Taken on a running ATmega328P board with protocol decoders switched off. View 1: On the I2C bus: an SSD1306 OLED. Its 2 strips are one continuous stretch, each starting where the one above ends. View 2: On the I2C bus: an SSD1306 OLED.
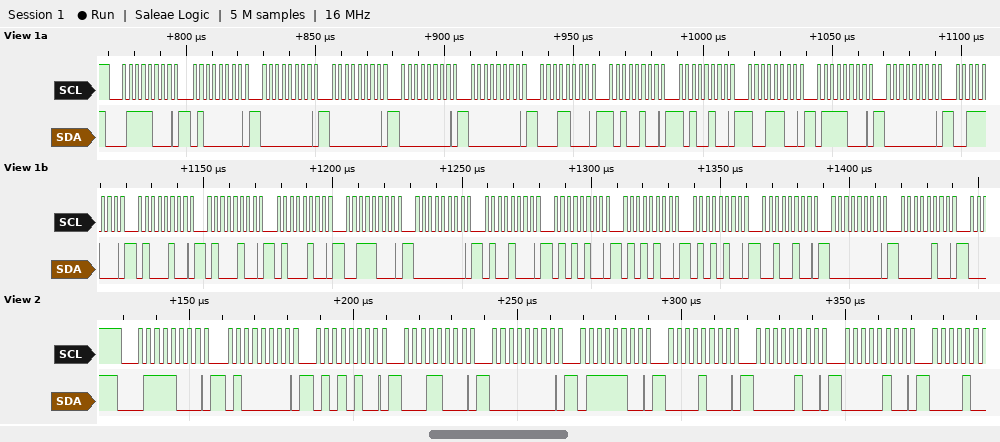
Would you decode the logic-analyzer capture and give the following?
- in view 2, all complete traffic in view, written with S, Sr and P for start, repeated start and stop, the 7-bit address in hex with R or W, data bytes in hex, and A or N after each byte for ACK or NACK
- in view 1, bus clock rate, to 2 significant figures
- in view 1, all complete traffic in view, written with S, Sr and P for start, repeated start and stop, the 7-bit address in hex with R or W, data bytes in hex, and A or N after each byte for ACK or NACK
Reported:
S 3CW A 40 A 54 A 18 A 00 A 7C A 08 A 04 A 04 A
400 kHz
S 3CW A 40 A 00 A 00 A 00 A 00 A 18 A A4 A A4 A 9C A 78 A 00 A 38 A 44 A 44 A 44 A 38 A 00 A 48 A 54 A 54 A 54 A 24 A 00 A 04 A
